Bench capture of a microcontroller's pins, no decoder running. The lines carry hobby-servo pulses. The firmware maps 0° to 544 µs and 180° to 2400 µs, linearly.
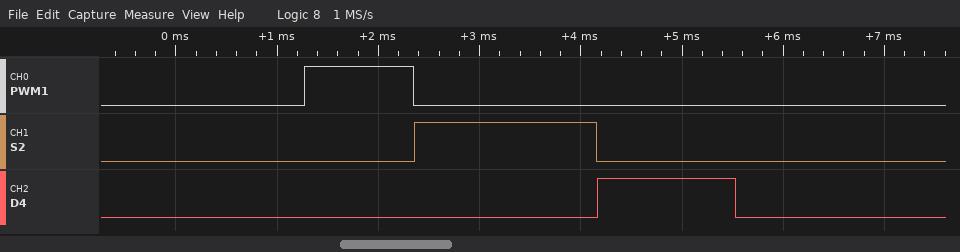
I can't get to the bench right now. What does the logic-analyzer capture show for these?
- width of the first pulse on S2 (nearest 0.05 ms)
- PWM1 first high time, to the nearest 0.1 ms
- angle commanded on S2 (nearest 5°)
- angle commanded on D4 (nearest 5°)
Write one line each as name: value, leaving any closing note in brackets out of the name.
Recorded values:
width of the first pulse on S2: 1.80 ms
PWM1 first high time, to the nearest 0.1 ms: 1.1 ms
angle commanded on S2: 120°
angle commanded on D4: 80°
